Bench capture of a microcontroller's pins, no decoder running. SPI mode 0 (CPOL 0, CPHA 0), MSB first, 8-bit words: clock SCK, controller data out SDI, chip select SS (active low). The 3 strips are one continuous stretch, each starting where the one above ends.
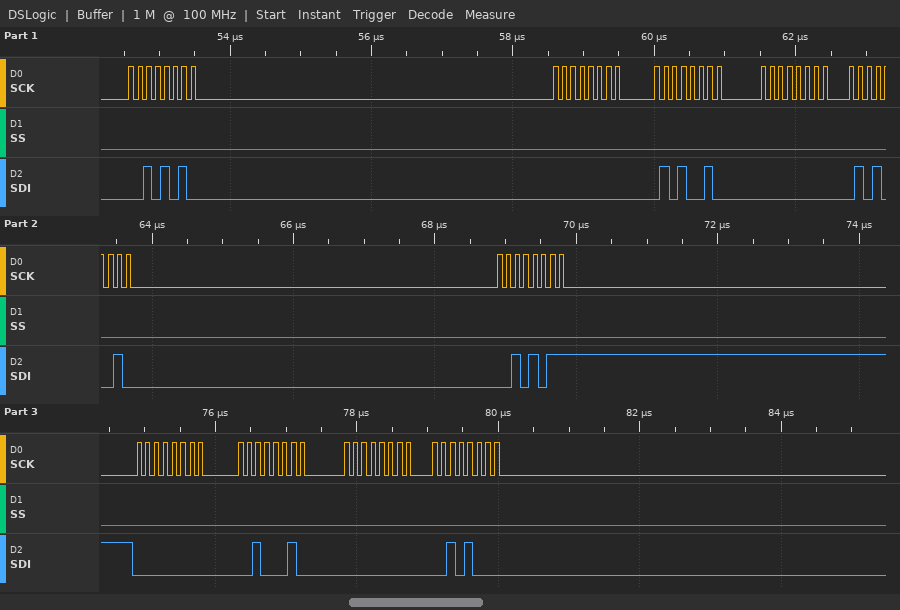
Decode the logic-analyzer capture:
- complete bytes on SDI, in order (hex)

2A 00 52 00 52 2B 00 22 00 28
